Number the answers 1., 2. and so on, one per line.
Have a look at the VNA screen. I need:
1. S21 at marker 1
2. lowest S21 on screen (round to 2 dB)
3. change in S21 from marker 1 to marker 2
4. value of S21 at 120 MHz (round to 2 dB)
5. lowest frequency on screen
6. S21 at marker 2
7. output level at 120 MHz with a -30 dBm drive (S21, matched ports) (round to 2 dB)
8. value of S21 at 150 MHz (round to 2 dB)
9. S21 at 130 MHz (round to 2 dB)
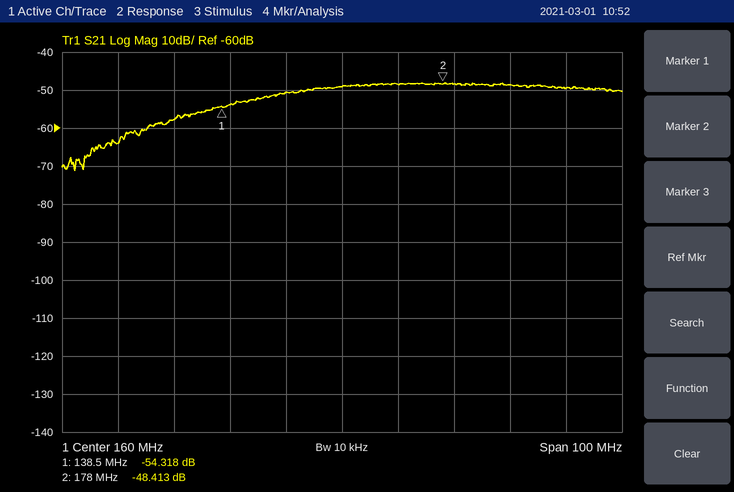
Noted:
1. -54.318 dB
2. -72 dB
3. 5.905 dB
4. -64 dB
5. 110 MHz
6. -48.413 dB
7. -94 dBm
8. -50 dB
9. -58 dB
